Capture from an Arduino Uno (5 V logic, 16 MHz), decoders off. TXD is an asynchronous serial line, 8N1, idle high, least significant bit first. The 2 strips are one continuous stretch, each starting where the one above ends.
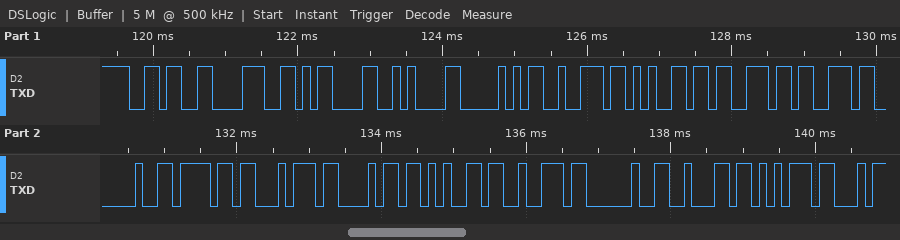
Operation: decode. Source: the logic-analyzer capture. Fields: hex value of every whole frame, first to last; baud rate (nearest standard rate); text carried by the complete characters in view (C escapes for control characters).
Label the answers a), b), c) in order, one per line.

a) 0x36 0x38 0x0D 0x0A 0x50 0x72 0x65 0x73 0x73 0x20 0x6F 0x74 0x68 0x65 0x72 0x20 0x62 0x75
b) 9600 baud
c) "68\r\nPress other bu"
